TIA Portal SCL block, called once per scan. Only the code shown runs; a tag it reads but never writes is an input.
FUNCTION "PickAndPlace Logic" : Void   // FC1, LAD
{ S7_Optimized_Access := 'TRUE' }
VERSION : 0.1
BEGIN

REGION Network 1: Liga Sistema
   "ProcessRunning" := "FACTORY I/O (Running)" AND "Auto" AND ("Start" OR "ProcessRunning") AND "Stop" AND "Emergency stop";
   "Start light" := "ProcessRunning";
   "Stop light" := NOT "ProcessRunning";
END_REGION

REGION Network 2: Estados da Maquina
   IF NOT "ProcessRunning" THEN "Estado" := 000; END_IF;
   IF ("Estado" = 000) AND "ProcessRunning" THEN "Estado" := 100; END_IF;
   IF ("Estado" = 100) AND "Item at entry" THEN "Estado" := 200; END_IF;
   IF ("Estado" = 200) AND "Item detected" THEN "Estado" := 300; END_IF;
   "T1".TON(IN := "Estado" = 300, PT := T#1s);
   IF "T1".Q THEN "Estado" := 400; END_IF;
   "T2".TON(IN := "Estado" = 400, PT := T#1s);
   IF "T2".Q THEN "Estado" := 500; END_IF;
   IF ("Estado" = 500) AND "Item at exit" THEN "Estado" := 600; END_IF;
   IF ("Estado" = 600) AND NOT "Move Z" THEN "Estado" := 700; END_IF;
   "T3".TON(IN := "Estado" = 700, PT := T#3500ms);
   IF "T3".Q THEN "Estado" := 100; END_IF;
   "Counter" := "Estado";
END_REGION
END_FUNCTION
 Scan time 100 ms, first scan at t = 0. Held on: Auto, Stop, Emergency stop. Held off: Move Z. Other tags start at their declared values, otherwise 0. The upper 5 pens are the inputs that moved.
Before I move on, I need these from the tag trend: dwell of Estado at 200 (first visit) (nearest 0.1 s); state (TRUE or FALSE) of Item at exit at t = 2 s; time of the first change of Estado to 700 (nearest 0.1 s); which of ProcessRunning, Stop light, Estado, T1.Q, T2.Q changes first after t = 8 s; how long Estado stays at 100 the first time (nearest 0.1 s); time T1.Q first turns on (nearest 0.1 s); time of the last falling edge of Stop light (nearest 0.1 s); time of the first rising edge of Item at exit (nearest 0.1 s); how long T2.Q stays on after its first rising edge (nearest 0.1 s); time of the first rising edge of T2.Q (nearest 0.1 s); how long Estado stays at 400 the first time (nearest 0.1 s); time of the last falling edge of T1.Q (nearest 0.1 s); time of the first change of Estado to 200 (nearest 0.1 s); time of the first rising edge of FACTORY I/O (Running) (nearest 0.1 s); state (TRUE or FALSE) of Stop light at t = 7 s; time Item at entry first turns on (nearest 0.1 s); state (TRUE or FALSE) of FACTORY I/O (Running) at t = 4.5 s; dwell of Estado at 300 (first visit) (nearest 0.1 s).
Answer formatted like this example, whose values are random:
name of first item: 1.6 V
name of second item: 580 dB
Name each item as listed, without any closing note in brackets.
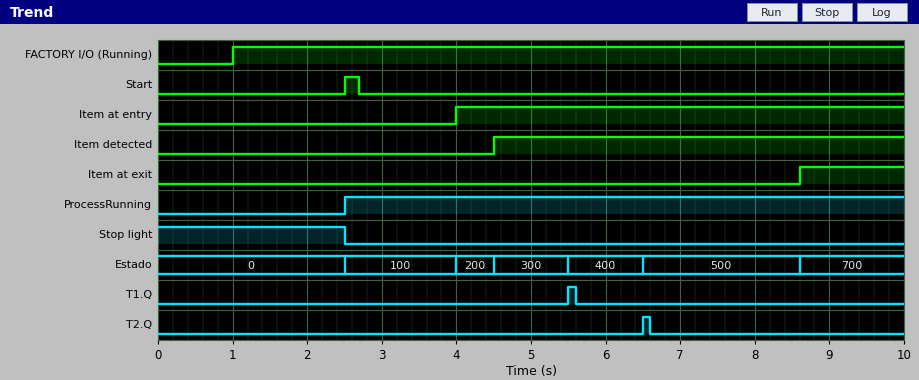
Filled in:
dwell of Estado at 200 (first visit): 0.5 s
state (TRUE or FALSE) of Item at exit at t = 2 s: FALSE
time of the first change of Estado to 700: 8.6 s
which of ProcessRunning, Stop light, Estado, T1.Q, T2.Q changes first after t = 8 s: Estado
how long Estado stays at 100 the first time: 1.5 s
time T1.Q first turns on: 5.5 s
time of the last falling edge of Stop light: 2.5 s
time of the first rising edge of Item at exit: 8.6 s
how long T2.Q stays on after its first rising edge: 0.1 s
time of the first rising edge of T2.Q: 6.5 s
how long Estado stays at 400 the first time: 1.0 s
time of the last falling edge of T1.Q: 5.6 s
time of the first change of Estado to 200: 4.0 s
time of the first rising edge of FACTORY I/O (Running): 1.0 s
state (TRUE or FALSE) of Stop light at t = 7 s: FALSE
time Item at entry first turns on: 4.0 s
state (TRUE or FALSE) of FACTORY I/O (Running) at t = 4.5 s: TRUE
dwell of Estado at 300 (first visit): 1.0 s
